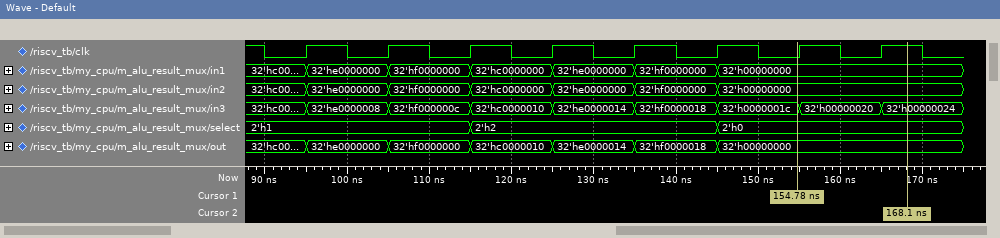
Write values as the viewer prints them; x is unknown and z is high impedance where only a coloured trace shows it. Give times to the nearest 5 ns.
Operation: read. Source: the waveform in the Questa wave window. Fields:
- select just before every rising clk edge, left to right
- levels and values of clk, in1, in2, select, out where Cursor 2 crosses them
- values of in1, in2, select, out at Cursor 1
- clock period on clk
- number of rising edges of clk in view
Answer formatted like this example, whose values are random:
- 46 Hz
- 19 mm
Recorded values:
- 2'h1, 2'h1, 2'h1, 2'h2, 2'h2, 2'h2, 2'h0, 2'h0
- clk=1, in1=32'h00000000, in2=32'h00000000, select=2'h0, out=32'h00000000
- in1=32'h00000000, in2=32'h00000000, select=2'h0, out=32'h00000000
- 10 ns
- 8
